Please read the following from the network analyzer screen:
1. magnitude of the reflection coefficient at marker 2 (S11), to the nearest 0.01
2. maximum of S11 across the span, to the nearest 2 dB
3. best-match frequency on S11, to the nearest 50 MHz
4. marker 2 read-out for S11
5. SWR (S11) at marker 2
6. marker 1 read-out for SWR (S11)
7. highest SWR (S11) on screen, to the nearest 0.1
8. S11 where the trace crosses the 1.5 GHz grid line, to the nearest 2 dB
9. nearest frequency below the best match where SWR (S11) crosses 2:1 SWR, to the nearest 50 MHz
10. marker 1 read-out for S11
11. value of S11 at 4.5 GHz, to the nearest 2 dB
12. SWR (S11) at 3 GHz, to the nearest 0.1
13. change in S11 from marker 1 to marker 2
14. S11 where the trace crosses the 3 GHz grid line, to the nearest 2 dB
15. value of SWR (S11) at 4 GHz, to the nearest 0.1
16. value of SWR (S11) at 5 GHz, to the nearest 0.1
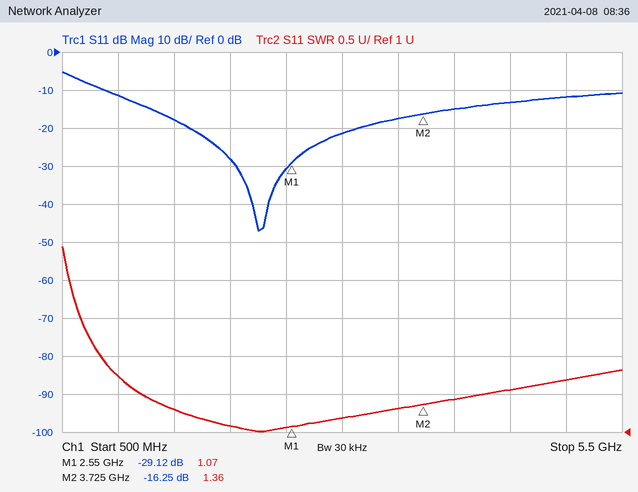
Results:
0.15
-6 dB
2.25 GHz
-16.25 dB
1.36
1.07
3.4
-18 dB
850 MHz
-29.12 dB
-14 dB
1.2
12.87 dB
-22 dB
1.4
1.7
